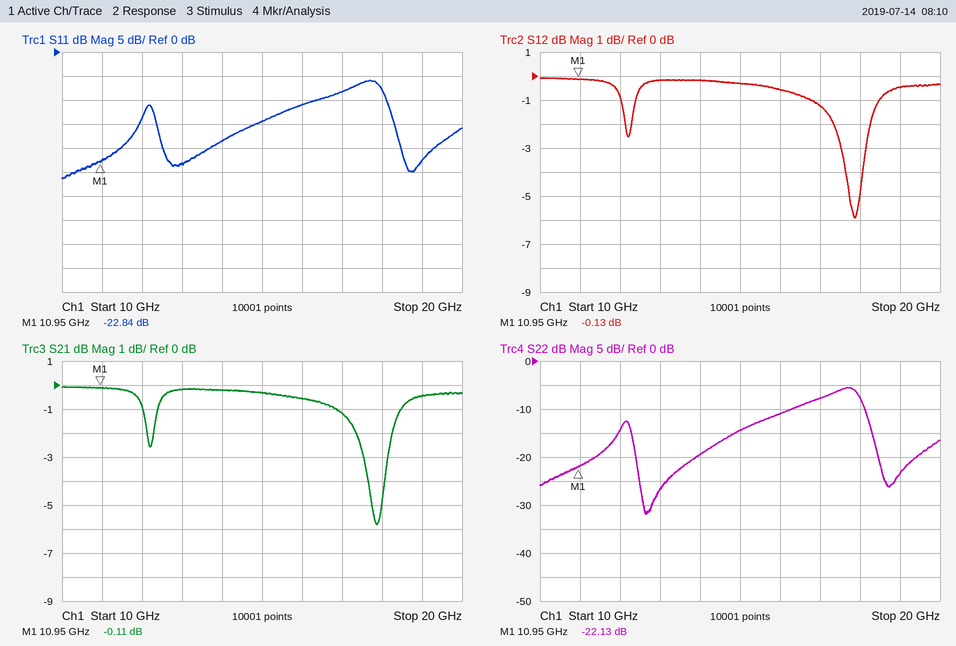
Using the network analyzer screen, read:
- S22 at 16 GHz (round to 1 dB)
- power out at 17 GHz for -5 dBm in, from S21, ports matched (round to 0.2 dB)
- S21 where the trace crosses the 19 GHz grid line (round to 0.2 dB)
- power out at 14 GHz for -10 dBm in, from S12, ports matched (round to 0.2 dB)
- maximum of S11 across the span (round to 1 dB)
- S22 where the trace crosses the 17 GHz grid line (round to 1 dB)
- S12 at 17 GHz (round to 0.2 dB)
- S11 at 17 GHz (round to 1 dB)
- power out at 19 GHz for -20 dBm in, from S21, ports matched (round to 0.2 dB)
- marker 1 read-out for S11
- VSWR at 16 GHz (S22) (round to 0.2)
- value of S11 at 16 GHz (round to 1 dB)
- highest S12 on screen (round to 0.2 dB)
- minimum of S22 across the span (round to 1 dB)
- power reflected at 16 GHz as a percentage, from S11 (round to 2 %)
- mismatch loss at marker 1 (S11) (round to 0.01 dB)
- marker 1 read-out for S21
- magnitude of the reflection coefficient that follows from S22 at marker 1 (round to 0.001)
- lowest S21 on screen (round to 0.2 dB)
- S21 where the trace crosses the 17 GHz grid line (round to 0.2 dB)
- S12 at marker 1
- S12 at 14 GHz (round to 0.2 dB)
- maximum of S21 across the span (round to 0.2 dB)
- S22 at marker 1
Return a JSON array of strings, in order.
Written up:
["-11 dB", "-6.2 dBm", "-0.4 dB", "-10.2 dBm", "-6 dB", "-8 dB", "-1.2 dB", "-8 dB", "-20.4 dBm", "-22.84 dB", "1.8", "-11 dB", "0.0 dB", "-32 dB", "8 %", "0.02 dB", "-0.11 dB", "0.078", "-5.8 dB", "-1.2 dB", "-0.13 dB", "-0.2 dB", "0.0 dB", "-22.13 dB"]
